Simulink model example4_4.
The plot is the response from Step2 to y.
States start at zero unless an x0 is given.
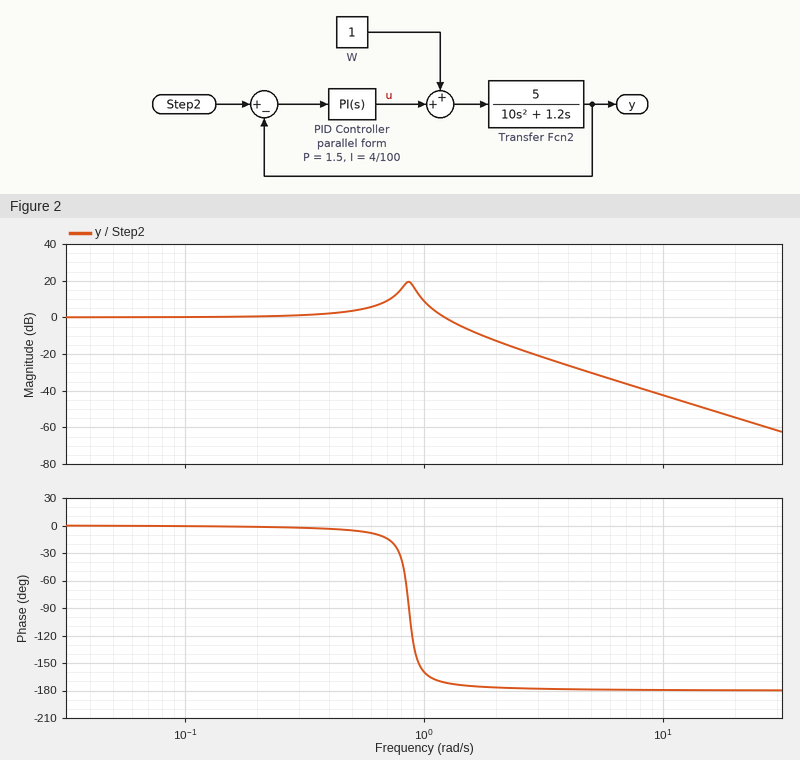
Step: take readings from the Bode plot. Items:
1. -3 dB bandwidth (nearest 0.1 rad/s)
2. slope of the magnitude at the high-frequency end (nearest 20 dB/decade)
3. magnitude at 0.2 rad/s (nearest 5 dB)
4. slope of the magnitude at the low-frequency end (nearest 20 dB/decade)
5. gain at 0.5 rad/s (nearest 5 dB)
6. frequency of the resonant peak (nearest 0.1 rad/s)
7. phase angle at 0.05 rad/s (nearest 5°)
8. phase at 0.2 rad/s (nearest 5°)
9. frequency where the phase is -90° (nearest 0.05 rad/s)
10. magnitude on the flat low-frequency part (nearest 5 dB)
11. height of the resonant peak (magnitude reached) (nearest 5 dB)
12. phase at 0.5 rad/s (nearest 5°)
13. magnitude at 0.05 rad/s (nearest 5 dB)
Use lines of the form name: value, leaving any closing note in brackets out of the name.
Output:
-3 dB bandwidth: 1.3 rad/s
slope of the magnitude at the high-frequency end: -40 dB/decade
magnitude at 0.2 rad/s: 0 dB
slope of the magnitude at the low-frequency end: 0 dB/decade
gain at 0.5 rad/s: 5 dB
frequency of the resonant peak: 0.9 rad/s
phase angle at 0.05 rad/s: 0°
phase at 0.2 rad/s: 0°
frequency where the phase is -90°: 0.85 rad/s
magnitude on the flat low-frequency part: 0 dB
height of the resonant peak (magnitude reached): 20 dB
phase at 0.5 rad/s: -5°
magnitude at 0.05 rad/s: 0 dB
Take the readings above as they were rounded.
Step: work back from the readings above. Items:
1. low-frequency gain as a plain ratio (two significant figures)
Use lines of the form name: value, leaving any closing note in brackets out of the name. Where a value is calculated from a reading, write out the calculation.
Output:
low-frequency gain as a plain ratio: 10^(0 / 20) = 1.0
